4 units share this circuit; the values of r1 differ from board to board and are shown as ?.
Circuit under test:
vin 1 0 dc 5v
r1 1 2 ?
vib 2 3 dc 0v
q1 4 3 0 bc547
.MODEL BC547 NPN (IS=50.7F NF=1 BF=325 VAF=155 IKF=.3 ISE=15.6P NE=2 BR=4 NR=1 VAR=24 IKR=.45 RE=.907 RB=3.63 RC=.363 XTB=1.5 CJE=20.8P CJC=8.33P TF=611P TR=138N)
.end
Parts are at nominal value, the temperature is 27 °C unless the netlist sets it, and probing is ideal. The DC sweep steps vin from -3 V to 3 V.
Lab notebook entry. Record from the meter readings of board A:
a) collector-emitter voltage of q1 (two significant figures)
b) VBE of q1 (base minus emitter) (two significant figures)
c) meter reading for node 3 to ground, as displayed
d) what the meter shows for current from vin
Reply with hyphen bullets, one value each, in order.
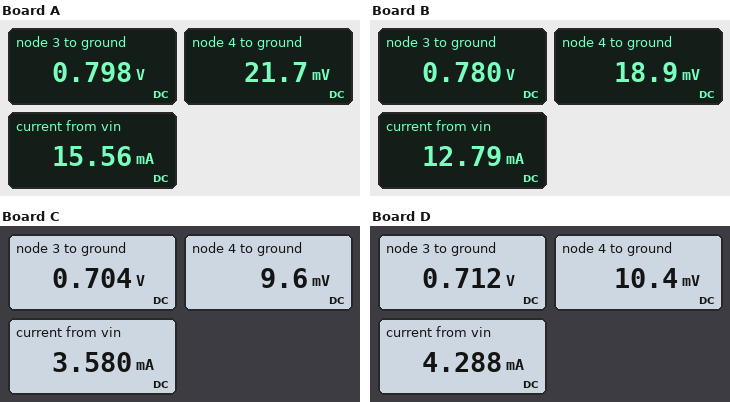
- 22 mV
- 800 mV
- 0.798 V
- 15.56 mA
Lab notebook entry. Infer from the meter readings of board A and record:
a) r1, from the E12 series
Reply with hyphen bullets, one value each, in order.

- 270 Ω
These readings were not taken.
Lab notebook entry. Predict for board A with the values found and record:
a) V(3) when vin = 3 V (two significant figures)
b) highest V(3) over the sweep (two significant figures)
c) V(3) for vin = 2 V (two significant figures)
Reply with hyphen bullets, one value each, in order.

- 750 mV
- 750 mV
- 720 mV
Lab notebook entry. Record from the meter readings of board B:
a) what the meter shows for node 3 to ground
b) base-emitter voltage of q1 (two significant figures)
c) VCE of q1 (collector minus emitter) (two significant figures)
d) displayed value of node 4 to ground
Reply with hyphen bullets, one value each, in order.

- 0.780 V
- 780 mV
- 19 mV
- 18.9 mV
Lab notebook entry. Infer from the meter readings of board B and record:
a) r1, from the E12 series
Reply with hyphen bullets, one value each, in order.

- 330 Ω
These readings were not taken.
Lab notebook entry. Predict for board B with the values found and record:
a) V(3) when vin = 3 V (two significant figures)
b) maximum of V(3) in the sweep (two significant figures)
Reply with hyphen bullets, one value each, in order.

- 740 mV
- 740 mV
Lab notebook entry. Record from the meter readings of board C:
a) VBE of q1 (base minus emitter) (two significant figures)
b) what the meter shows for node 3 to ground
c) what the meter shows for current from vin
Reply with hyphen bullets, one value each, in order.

- 700 mV
- 0.704 V
- 3.580 mA
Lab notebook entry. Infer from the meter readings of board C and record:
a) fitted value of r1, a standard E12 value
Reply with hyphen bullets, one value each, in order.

- 1.2 kΩ
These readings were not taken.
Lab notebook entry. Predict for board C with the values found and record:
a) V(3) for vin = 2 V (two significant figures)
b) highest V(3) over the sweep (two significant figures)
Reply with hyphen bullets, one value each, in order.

- 660 mV
- 680 mV
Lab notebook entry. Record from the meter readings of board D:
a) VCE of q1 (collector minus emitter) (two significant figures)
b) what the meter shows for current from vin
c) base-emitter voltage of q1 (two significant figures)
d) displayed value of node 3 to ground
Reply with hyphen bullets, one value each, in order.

- 10 mV
- 4.288 mA
- 710 mV
- 0.712 V
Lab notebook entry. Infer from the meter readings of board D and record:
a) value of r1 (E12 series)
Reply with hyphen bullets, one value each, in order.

- 1 kΩ
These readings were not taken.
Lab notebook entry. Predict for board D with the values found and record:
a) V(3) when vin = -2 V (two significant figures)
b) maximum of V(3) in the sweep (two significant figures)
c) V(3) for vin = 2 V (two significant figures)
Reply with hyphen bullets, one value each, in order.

- -2.0 V
- 690 mV
- 670 mV
